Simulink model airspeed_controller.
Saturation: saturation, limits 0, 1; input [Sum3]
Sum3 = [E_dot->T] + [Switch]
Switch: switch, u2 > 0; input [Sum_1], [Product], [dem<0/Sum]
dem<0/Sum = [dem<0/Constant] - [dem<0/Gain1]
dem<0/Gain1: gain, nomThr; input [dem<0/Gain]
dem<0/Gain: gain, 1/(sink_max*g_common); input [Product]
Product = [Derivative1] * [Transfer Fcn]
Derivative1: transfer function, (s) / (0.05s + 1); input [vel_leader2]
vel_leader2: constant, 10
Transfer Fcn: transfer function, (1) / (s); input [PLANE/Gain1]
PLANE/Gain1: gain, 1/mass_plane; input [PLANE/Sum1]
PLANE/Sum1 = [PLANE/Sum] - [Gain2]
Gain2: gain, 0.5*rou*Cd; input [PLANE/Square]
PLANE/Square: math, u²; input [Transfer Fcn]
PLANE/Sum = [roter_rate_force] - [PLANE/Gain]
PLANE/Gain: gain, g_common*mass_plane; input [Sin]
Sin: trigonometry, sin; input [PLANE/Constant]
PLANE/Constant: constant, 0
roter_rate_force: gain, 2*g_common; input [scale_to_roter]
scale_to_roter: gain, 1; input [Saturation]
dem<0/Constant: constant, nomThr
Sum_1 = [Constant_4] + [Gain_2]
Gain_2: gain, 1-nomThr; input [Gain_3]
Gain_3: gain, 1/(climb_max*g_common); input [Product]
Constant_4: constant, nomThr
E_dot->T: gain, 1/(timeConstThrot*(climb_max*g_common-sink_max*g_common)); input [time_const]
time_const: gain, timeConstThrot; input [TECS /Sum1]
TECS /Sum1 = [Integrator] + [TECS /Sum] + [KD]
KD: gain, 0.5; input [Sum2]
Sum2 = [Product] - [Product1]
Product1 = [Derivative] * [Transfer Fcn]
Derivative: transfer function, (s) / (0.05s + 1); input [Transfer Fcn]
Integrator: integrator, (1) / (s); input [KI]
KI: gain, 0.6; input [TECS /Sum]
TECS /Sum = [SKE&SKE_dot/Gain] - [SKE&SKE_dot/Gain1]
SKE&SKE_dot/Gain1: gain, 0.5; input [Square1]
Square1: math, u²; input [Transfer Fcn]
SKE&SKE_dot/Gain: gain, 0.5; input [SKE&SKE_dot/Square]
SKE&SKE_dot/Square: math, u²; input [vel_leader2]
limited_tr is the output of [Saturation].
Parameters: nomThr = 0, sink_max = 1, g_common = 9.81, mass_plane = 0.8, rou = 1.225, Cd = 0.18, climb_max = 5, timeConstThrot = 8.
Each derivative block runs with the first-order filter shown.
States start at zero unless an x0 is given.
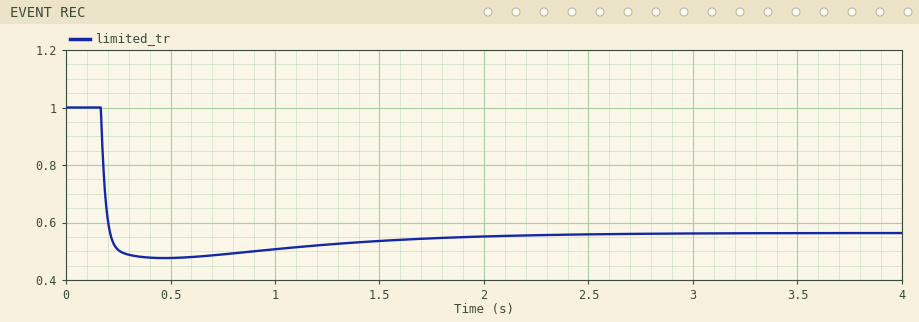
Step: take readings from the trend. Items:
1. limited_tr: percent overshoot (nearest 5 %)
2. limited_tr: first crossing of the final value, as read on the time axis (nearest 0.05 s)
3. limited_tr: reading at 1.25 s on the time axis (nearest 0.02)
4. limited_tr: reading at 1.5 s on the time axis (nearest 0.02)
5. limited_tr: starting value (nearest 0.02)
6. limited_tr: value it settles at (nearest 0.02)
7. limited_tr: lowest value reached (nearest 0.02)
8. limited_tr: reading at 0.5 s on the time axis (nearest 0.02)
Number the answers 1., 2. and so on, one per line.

1. 20 %
2. 0.20 s
3. 0.52
4. 0.54
5. 1.00
6. 0.56
7. 0.48
8. 0.48
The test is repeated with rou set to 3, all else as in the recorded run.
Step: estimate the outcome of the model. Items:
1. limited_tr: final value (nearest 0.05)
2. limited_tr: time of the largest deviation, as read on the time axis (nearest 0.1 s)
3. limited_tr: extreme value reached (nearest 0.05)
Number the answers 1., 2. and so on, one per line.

1. 1.00
2. 0.3 s
3. 0.65
